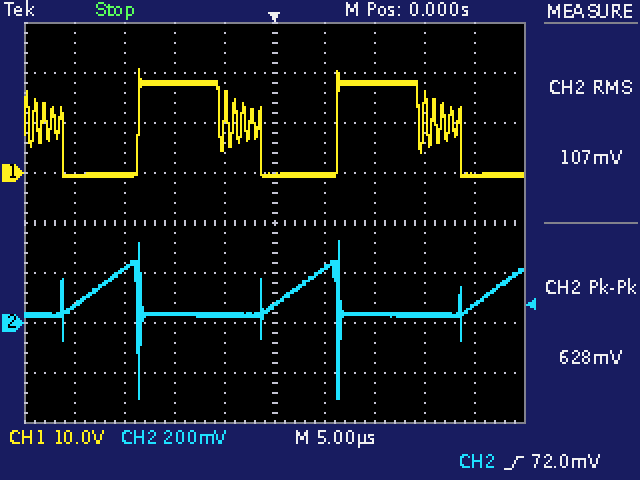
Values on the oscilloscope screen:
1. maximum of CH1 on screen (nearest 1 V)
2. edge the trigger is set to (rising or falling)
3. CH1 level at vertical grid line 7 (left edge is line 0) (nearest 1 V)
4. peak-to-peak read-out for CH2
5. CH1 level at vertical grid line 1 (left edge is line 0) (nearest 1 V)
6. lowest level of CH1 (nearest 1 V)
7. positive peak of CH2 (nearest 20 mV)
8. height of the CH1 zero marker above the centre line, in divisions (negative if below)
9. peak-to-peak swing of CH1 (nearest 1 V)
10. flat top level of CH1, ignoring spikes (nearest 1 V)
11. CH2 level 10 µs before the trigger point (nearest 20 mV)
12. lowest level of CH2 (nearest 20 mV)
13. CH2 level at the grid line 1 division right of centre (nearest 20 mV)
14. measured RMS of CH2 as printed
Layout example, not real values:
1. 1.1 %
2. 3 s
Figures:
1. 21 V
2. rising
3. 18 V
4. 628 mV
5. -1 V
6. -1 V
7. 320 mV
8. +1.0 div
9. 22 V
10. 18 V
11. 40 mV
12. -300 mV
13. 220 mV
14. 107 mV
